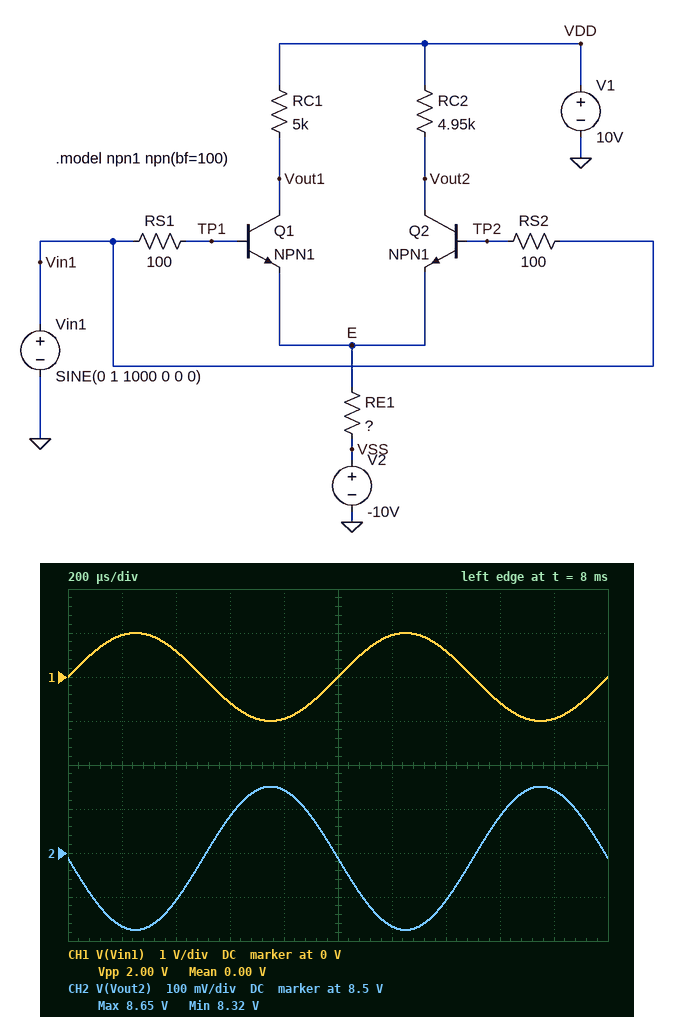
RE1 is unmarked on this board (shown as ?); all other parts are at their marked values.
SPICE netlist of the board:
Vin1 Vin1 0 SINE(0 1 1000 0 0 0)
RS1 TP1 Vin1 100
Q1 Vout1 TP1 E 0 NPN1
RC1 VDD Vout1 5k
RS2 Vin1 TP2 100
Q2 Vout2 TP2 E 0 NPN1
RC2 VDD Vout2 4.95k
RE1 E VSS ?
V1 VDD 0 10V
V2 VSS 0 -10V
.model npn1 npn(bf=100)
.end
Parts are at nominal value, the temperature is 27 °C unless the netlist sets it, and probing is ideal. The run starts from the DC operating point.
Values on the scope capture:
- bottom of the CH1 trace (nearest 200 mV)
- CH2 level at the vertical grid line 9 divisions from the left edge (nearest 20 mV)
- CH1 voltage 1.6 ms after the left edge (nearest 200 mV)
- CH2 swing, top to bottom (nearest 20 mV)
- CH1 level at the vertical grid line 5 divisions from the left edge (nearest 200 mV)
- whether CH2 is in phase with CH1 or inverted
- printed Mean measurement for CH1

-1.0 V
8.64 V
-600 mV
320 mV
0 V
inverted
0.00 V
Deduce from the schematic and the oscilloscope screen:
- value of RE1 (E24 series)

15 kΩ
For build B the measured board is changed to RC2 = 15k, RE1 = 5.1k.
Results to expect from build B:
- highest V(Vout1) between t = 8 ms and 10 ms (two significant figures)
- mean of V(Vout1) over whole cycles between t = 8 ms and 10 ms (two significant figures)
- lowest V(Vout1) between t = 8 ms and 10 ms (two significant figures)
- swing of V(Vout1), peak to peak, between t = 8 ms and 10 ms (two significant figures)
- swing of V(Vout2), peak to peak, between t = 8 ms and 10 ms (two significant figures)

5.9 V
4.9 V
3.8 V
2.1 V
1.9 V
